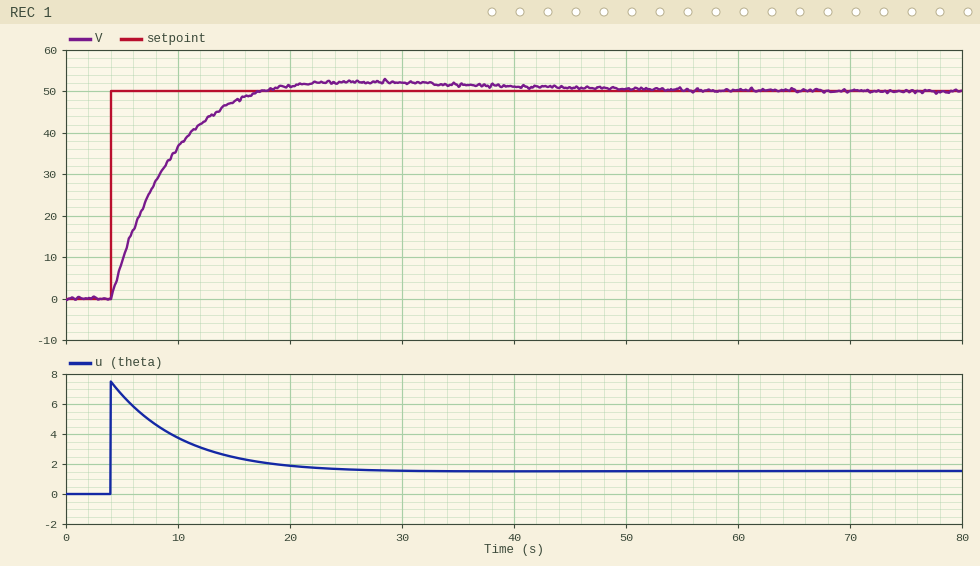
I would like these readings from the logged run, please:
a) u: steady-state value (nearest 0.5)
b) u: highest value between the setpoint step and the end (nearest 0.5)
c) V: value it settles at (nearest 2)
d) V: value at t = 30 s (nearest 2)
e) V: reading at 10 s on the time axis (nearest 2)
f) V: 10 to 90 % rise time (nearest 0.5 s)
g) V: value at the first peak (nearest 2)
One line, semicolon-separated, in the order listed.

1.5; 7.5; 50; 52; 36; 9.0 s; 52
